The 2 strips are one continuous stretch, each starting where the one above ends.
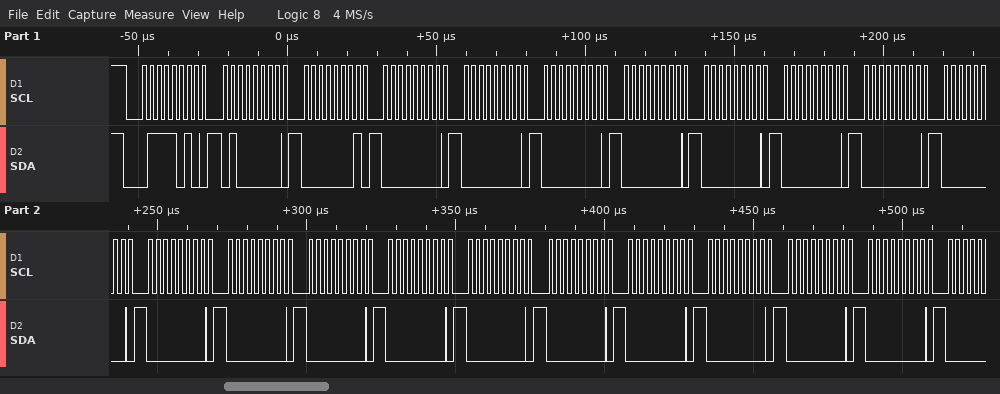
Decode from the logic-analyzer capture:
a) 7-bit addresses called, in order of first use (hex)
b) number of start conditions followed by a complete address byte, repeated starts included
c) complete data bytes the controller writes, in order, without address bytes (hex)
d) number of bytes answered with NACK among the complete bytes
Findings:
0x3D
1
40 01 00 00 00 00 00 00 00 00 00 00 00 00 00 00 00 00 00 00
0
